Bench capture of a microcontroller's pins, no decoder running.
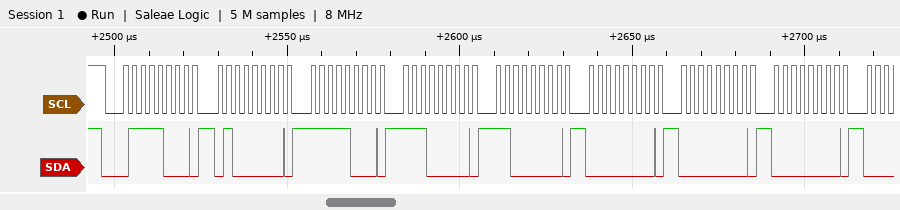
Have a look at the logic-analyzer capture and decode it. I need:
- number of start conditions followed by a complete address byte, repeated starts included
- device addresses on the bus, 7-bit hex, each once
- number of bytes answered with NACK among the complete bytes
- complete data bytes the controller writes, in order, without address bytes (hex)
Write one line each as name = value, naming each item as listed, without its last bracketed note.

number of start conditions followed by a complete address byte, repeated starts included = 1
device addresses on the bus, 7-bit hex, each once = 0x3C
number of bytes answered with NACK among the complete bytes = 0
complete data bytes the controller writes, in order, without address bytes = 40 F8 E0 C0 00 00 00
